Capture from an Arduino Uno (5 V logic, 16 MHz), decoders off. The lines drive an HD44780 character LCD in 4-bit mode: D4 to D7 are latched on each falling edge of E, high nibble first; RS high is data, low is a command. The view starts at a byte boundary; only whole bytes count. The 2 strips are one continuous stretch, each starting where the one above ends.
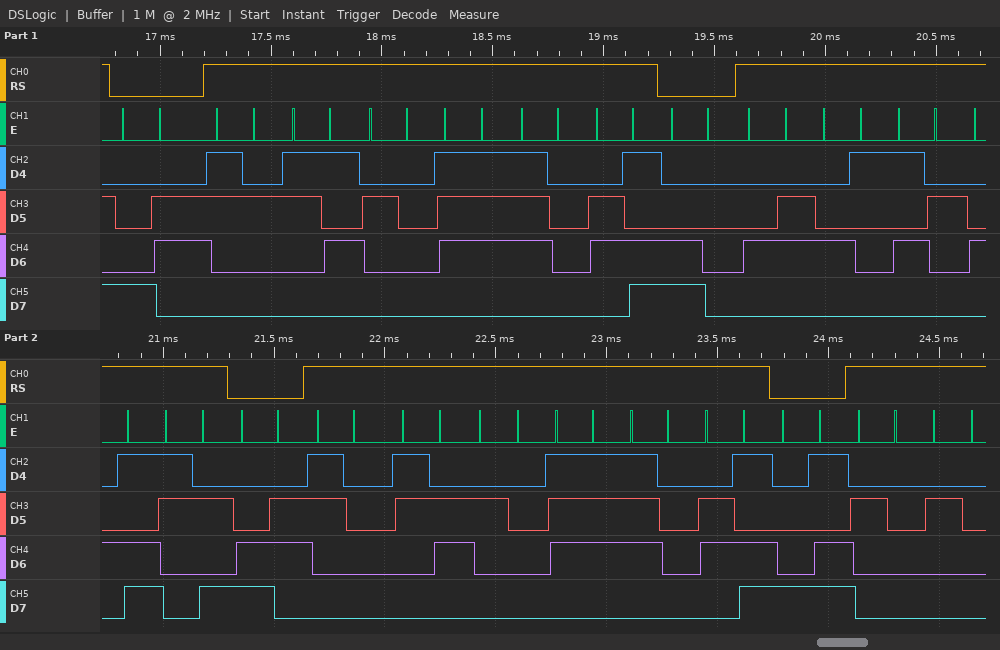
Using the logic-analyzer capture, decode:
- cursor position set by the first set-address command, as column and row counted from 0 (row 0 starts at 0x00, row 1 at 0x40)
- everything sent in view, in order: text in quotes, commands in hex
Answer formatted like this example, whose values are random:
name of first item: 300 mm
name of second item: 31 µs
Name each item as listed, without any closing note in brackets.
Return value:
cursor position set by the first set-address command, as column and row counted from 0: column 6, row 0
everything sent in view, in order: text in quotes, commands in hex: 0x86 "25 wpm" 0xC0 "FARM:" 0xC6 "06 wpm" 0x8D "  "
